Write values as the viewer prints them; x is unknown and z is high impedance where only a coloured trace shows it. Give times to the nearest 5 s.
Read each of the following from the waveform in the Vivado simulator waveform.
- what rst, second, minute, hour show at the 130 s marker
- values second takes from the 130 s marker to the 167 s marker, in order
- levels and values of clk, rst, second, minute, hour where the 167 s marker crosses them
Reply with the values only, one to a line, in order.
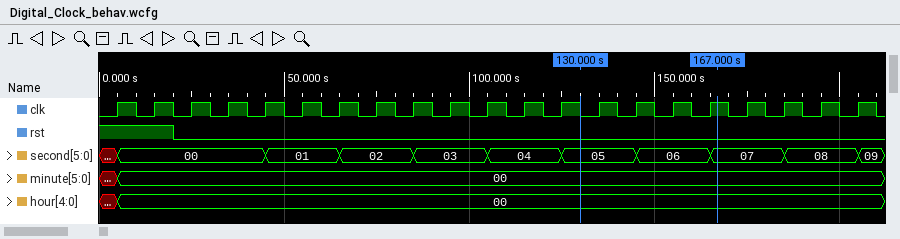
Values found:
rst=0, second=05, minute=00, hour=00
05, 06, 07
clk=1, rst=0, second=07, minute=00, hour=00
